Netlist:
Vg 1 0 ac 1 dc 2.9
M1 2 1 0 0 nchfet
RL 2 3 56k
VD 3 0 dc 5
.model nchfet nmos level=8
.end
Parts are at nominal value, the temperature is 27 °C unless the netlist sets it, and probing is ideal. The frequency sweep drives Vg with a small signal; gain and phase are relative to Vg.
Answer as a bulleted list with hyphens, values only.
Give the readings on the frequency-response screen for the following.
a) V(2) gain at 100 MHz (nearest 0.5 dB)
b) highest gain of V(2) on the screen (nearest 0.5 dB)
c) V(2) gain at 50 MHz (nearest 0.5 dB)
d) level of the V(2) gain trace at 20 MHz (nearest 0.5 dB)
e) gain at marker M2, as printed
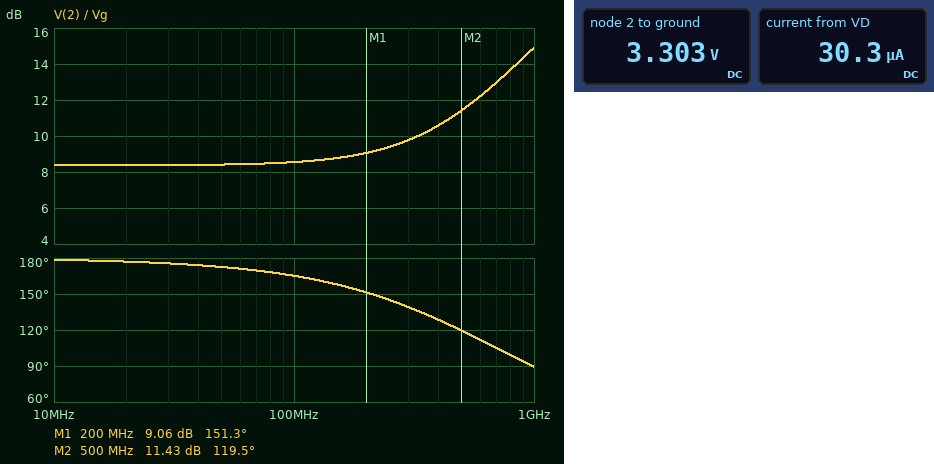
- 8.5 dB
- 15.0 dB
- 8.5 dB
- 8.5 dB
- 11.43 dB
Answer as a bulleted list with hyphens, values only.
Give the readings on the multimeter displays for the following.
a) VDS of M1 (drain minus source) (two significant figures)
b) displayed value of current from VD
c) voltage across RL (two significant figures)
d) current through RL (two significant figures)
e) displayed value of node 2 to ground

- 3.3 V
- 30.3 µA
- 1.7 V
- 30 µA
- 3.303 V
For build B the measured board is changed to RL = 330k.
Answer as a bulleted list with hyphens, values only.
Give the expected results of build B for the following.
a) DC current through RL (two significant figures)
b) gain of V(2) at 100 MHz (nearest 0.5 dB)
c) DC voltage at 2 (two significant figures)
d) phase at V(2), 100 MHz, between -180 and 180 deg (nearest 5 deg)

- 15 µA
- -10.5 dB
- 180 mV
- 110 deg
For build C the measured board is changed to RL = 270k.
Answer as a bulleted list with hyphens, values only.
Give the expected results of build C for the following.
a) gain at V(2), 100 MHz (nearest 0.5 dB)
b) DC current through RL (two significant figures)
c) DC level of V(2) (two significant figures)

- -8.5 dB
- 18 µA
- 220 mV
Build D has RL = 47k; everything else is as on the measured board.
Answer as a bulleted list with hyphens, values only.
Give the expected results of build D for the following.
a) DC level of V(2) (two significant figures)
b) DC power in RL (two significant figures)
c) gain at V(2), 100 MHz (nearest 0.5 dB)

- 3.6 V
- 43 µW
- 7.0 dB
